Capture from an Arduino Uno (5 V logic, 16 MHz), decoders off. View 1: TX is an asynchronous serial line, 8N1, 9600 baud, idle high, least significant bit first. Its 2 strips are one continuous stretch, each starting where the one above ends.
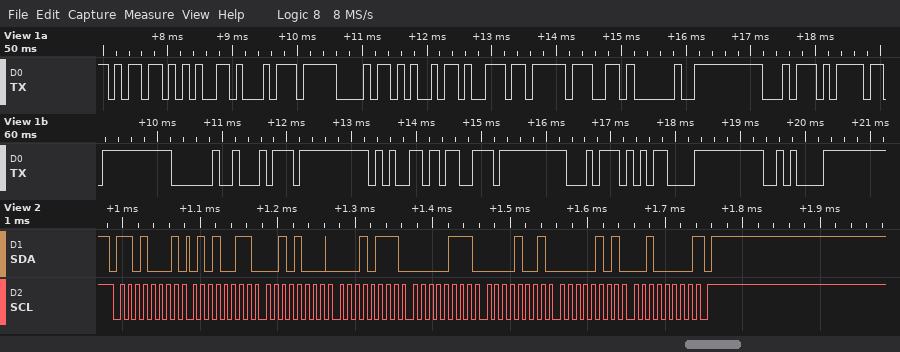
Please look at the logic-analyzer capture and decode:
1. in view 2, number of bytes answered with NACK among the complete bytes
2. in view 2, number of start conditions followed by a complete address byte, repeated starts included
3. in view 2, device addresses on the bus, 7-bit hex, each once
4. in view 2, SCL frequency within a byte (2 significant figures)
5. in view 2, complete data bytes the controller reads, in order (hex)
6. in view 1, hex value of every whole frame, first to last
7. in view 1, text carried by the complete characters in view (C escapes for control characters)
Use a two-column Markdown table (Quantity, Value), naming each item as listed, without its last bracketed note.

| Quantity | Value |
|---|---|
| in view 2, number of bytes answered with NACK among the complete bytes | 1 |
| in view 2, number of start conditions followed by a complete address byte, repeated starts included | 1 |
| in view 2, device addresses on the bus, 7-bit hex, each once | 0x68 |
| in view 2, SCL frequency within a byte | 100 kHz |
| in view 2, complete data bytes the controller reads, in order | 53 28 17 07 09 05 20 |
| in view 1, hex value of every whole frame, first to last | 6D 65 74 68 69 6E 67 20 74 6F 20 74 65 73 74 0D 0A |
| in view 1, text carried by the complete characters in view | "mething to test\r\n" |
